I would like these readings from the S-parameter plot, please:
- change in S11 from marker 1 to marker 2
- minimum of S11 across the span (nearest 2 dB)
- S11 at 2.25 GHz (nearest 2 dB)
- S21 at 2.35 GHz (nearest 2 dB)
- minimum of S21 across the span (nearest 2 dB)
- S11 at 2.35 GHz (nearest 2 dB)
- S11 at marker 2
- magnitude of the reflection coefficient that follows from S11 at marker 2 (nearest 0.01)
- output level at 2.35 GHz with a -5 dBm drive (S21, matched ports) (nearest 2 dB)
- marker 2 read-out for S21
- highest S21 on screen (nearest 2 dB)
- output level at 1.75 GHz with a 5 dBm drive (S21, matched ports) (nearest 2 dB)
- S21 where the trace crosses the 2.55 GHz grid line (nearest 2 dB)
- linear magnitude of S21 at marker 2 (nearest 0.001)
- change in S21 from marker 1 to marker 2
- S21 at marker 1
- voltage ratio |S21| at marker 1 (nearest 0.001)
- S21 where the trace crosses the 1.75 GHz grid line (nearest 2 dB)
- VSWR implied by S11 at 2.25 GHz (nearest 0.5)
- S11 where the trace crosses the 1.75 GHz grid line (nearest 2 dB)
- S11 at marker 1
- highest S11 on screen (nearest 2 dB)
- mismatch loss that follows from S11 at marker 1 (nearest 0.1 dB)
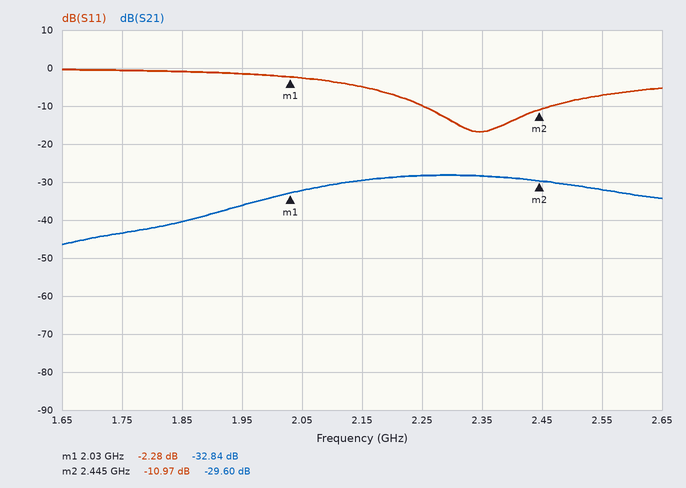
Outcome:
-8.69 dB
-16 dB
-10 dB
-28 dB
-46 dB
-16 dB
-10.97 dB
0.28
-34 dBm
-29.60 dB
-28 dB
-38 dBm
-32 dB
0.033
3.24 dB
-32.84 dB
0.023
-44 dB
2.0
0 dB
-2.28 dB
0 dB
3.9 dB
